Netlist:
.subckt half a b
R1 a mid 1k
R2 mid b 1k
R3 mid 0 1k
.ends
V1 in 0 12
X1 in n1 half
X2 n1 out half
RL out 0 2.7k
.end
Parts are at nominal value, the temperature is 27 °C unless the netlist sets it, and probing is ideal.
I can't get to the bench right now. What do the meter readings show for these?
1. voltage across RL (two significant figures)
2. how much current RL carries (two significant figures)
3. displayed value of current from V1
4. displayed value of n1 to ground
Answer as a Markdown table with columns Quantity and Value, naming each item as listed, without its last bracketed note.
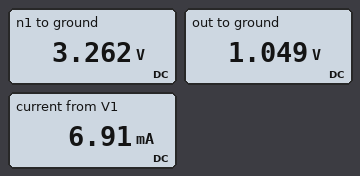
| Quantity | Value |
|---|---|
| voltage across RL | 1.0 V |
| how much current RL carries | 390 µA |
| displayed value of current from V1 | 6.91 mA |
| displayed value of n1 to ground | 3.262 V |
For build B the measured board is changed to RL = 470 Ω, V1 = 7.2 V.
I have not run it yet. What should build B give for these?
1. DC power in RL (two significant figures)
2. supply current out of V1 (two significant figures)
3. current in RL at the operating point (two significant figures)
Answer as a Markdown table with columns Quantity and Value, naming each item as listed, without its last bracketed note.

| Quantity | Value |
|---|---|
| DC power in RL | 100 µW |
| supply current out of V1 | 4.2 mA |
| current in RL at the operating point | 470 µA |
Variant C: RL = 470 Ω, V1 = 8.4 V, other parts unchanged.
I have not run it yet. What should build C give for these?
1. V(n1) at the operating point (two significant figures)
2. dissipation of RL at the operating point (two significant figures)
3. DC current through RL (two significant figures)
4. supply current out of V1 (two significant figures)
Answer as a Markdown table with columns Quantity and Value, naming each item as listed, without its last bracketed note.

| Quantity | Value |
|---|---|
| V(n1) at the operating point | 2.2 V |
| dissipation of RL at the operating point | 140 µW |
| DC current through RL | 550 µA |
| supply current out of V1 | 4.9 mA |
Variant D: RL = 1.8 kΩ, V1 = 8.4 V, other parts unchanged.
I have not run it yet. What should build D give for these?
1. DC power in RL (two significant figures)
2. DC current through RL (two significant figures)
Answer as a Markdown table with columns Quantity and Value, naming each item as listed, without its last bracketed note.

| Quantity | Value |
|---|---|
| DC power in RL | 210 µW |
| DC current through RL | 340 µA |
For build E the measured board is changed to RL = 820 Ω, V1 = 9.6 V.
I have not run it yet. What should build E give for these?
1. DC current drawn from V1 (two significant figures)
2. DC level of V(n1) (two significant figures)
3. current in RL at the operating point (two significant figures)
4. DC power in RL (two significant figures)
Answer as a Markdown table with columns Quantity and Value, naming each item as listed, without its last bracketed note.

| Quantity | Value |
|---|---|
| DC current drawn from V1 | 5.6 mA |
| DC level of V(n1) | 2.5 V |
| current in RL at the operating point | 540 µA |
| DC power in RL | 240 µW |
